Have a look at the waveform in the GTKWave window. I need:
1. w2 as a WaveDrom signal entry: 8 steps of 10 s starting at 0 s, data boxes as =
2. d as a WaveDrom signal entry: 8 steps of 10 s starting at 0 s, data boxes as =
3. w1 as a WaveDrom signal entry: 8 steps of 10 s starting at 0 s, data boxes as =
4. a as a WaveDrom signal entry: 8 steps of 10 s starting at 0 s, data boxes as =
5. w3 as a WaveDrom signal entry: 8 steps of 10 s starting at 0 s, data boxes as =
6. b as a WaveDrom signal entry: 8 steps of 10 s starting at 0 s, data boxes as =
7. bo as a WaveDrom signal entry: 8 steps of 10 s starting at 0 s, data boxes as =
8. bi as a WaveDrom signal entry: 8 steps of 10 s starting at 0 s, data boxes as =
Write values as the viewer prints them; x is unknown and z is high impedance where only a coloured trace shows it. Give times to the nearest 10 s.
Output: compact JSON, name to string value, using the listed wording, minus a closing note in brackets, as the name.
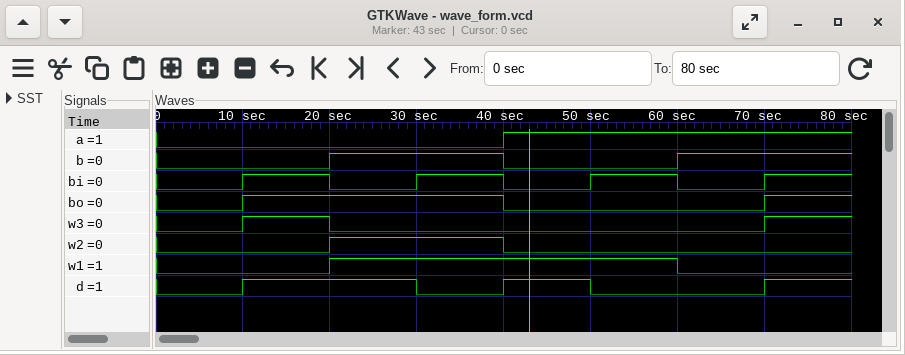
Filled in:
{"w2 as a WaveDrom signal entry: 8 steps of 10 s starting at 0 s, data boxes as =": "{name: 'w2', wave: '0.1.0...'}", "d as a WaveDrom signal entry: 8 steps of 10 s starting at 0 s, data boxes as =": "{name: 'd', wave: '01.010.1'}", "w1 as a WaveDrom signal entry: 8 steps of 10 s starting at 0 s, data boxes as =": "{name: 'w1', wave: '0.1...0.'}", "a as a WaveDrom signal entry: 8 steps of 10 s starting at 0 s, data boxes as =": "{name: 'a', wave: '0...1...'}", "w3 as a WaveDrom signal entry: 8 steps of 10 s starting at 0 s, data boxes as =": "{name: 'w3', wave: '010....1'}", "b as a WaveDrom signal entry: 8 steps of 10 s starting at 0 s, data boxes as =": "{name: 'b', wave: '0.1.0.1.'}", "bo as a WaveDrom signal entry: 8 steps of 10 s starting at 0 s, data boxes as =": "{name: 'bo', wave: '01..0..1'}", "bi as a WaveDrom signal entry: 8 steps of 10 s starting at 0 s, data boxes as =": "{name: 'bi', wave: '01010101'}"}
